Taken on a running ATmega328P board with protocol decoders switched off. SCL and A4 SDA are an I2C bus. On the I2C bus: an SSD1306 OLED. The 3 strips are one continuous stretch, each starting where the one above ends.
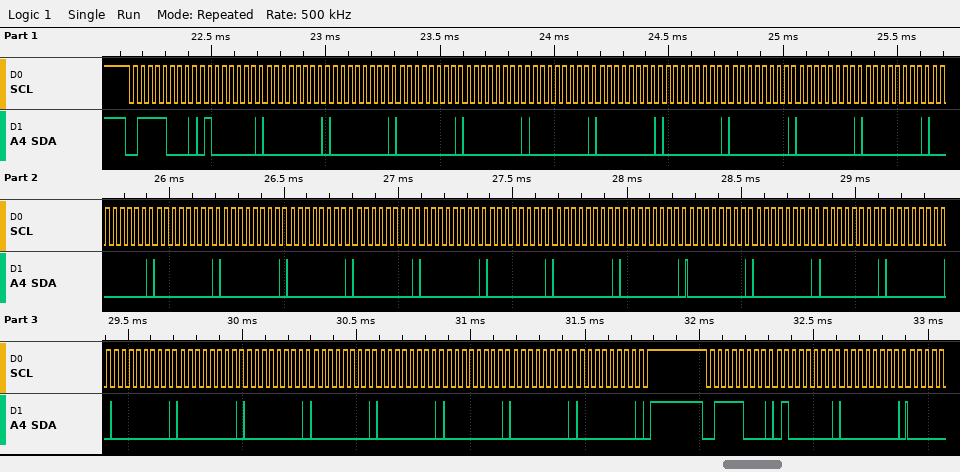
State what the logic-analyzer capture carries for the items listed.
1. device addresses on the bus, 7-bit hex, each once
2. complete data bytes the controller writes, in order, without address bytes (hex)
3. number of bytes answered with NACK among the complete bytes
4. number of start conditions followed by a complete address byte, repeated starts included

0x3C
40 00 00 00 00 00 00 00 00 00 00 00 00 00 00 00 00 00 00 00 00 00 00 00 00 00 00 00 00 00 00 00 40 00
0
2
